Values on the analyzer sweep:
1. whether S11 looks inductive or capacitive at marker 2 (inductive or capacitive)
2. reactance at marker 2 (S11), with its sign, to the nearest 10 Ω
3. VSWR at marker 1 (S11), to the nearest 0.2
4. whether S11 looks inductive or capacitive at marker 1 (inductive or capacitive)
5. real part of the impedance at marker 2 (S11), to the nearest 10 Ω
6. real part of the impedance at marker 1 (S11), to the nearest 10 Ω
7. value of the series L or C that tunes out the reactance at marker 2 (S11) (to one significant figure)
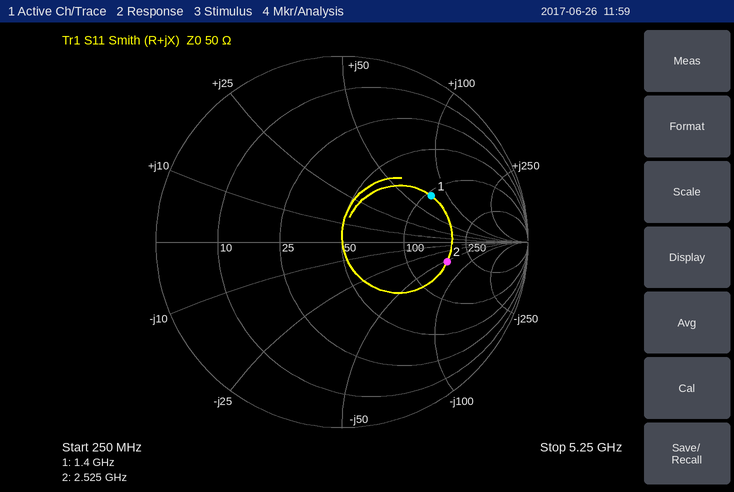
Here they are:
capacitive
-50 Ω
3.4
inductive
170 Ω
110 Ω
3 nH
